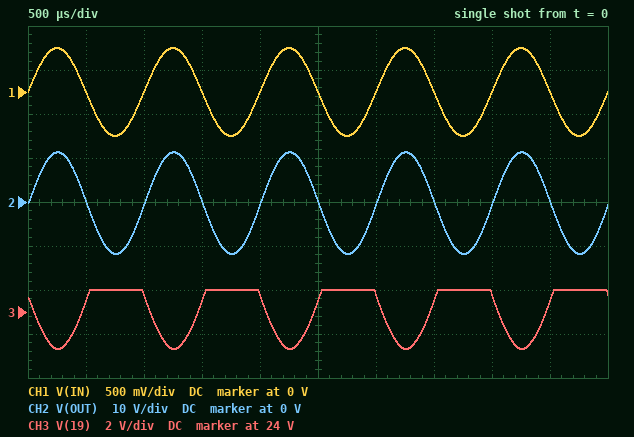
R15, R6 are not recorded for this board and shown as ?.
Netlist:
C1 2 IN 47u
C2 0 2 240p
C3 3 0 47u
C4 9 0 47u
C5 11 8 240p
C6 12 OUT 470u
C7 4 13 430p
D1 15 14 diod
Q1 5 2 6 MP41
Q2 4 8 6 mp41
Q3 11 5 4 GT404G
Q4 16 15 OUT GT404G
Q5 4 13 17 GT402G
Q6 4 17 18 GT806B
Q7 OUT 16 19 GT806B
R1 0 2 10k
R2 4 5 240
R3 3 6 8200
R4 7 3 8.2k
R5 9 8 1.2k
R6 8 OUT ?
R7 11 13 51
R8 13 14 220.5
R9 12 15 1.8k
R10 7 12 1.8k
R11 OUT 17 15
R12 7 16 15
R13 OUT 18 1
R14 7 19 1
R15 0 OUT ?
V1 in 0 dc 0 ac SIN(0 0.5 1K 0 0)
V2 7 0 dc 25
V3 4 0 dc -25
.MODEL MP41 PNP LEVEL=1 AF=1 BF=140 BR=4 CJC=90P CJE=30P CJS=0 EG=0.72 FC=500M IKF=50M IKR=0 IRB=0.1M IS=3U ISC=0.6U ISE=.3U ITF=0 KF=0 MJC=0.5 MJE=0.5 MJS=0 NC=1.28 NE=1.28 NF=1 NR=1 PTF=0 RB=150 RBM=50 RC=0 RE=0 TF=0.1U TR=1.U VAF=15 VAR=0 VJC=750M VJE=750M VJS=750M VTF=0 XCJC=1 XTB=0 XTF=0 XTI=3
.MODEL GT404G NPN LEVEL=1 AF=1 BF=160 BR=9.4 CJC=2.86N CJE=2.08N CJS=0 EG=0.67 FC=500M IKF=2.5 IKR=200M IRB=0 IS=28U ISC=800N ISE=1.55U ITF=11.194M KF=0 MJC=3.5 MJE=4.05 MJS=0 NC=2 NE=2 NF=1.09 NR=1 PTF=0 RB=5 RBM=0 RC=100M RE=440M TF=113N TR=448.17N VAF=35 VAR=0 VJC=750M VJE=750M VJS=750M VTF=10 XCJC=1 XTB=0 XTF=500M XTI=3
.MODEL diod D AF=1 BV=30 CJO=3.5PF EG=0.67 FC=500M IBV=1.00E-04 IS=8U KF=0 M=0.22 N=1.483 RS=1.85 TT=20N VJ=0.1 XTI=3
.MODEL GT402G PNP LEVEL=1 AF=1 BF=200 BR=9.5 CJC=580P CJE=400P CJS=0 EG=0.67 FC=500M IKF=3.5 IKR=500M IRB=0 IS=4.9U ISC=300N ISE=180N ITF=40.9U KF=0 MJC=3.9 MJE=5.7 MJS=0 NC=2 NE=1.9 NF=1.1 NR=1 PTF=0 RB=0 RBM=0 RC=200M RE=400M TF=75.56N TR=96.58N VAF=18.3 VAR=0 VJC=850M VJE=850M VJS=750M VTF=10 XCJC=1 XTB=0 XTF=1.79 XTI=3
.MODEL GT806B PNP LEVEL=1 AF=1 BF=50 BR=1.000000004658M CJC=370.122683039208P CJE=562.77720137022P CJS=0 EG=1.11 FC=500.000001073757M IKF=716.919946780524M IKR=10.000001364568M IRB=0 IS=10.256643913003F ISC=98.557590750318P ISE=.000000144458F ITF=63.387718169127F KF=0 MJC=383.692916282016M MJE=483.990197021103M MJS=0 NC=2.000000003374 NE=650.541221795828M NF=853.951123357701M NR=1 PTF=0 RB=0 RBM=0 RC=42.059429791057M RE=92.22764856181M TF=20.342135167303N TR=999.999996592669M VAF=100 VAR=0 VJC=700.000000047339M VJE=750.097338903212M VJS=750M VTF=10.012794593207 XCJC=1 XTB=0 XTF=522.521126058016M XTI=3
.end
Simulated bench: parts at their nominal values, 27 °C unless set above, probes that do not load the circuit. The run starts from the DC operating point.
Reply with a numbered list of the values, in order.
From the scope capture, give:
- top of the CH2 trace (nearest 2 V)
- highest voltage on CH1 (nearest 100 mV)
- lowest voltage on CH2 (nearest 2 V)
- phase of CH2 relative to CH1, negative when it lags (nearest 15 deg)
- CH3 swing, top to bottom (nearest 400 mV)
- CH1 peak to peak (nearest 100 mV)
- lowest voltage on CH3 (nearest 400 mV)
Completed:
1. 12 V
2. 500 mV
3. -12 V
4. 0 deg
5. 2.8 V
6. 1.0 V
7. 22.4 V
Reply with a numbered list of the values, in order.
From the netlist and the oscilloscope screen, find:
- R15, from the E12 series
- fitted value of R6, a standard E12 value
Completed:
1. 3.9 Ω
2. 27 kΩ
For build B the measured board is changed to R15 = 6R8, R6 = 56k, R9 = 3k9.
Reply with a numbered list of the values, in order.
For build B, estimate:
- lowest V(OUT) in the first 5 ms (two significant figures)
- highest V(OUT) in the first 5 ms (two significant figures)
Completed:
1. -20 V
2. 21 V
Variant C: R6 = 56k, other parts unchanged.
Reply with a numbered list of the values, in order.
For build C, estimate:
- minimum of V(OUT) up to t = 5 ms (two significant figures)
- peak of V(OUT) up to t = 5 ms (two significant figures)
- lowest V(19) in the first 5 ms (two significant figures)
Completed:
1. -18 V
2. 17 V
3. 21 V
